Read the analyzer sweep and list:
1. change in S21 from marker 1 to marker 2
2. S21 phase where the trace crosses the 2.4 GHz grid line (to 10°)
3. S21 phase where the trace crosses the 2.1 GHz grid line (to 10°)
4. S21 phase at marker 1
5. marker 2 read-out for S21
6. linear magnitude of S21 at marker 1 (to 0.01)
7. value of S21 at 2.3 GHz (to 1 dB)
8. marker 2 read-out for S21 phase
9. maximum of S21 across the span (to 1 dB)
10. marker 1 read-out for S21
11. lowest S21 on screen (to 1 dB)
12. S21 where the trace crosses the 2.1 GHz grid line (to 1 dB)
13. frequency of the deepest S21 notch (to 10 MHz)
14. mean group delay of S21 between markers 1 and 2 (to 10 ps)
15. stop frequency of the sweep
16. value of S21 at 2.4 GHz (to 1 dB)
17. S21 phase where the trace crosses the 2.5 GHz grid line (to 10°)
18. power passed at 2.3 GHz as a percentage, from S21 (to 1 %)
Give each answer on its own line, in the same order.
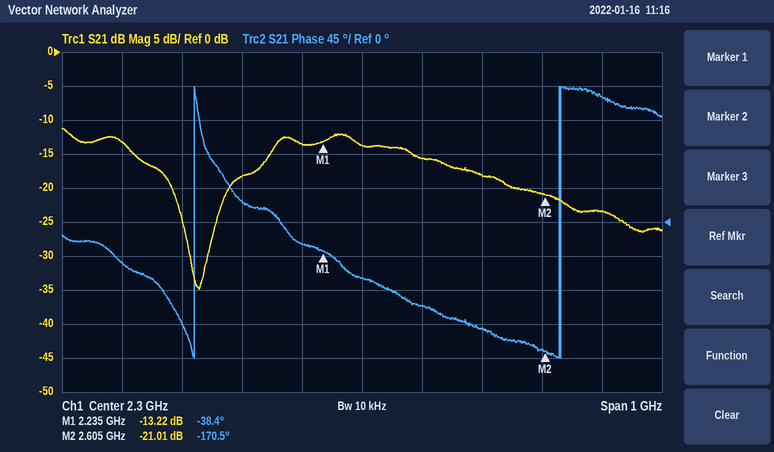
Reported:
-7.79 dB
-110°
30°
-38.4°
-21.01 dB
0.22
-14 dB
-170.5°
-11 dB
-13.22 dB
-35 dB
-18 dB
2.03 GHz
990 ps
2.8 GHz
-16 dB
-140°
4 %
